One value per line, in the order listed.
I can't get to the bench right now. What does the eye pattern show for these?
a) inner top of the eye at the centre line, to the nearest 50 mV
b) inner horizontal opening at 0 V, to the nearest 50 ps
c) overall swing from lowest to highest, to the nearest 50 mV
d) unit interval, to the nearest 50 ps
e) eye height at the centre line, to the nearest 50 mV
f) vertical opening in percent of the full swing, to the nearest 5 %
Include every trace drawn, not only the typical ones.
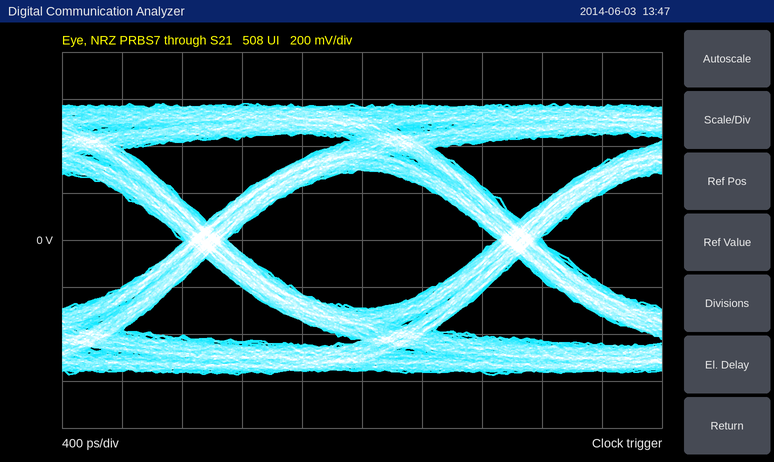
300 mV
1.80 ns
1.15 V
2.10 ns
600 mV
50 %
